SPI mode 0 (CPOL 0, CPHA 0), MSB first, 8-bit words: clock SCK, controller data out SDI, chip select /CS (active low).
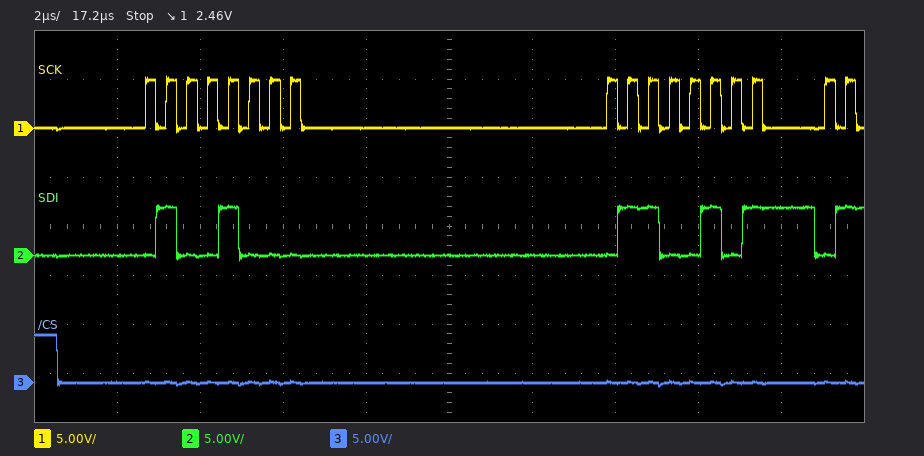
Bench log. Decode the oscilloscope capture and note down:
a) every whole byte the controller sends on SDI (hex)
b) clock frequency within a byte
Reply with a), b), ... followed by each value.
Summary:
a) 48 65
b) 2 MHz
